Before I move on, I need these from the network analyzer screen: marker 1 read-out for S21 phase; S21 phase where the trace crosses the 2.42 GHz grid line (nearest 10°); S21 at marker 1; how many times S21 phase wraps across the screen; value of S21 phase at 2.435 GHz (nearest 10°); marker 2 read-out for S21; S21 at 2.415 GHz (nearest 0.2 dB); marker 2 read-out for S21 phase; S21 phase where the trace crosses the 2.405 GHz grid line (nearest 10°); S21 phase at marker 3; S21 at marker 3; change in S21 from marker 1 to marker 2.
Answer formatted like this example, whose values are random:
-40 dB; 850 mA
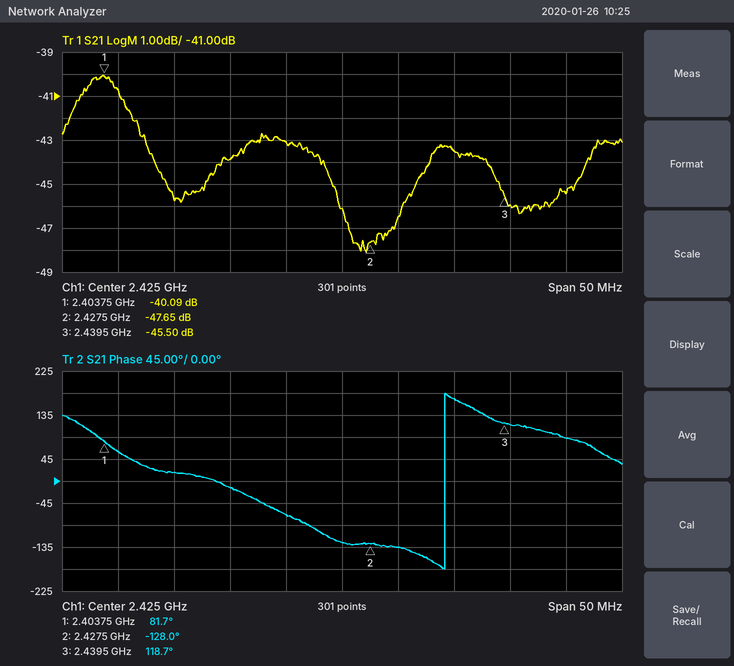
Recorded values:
81.7°; -70°; -40.09 dB; 1; 170°; -47.65 dB; -43.8 dB; -128.0°; 60°; 118.7°; -45.50 dB; -7.56 dB
